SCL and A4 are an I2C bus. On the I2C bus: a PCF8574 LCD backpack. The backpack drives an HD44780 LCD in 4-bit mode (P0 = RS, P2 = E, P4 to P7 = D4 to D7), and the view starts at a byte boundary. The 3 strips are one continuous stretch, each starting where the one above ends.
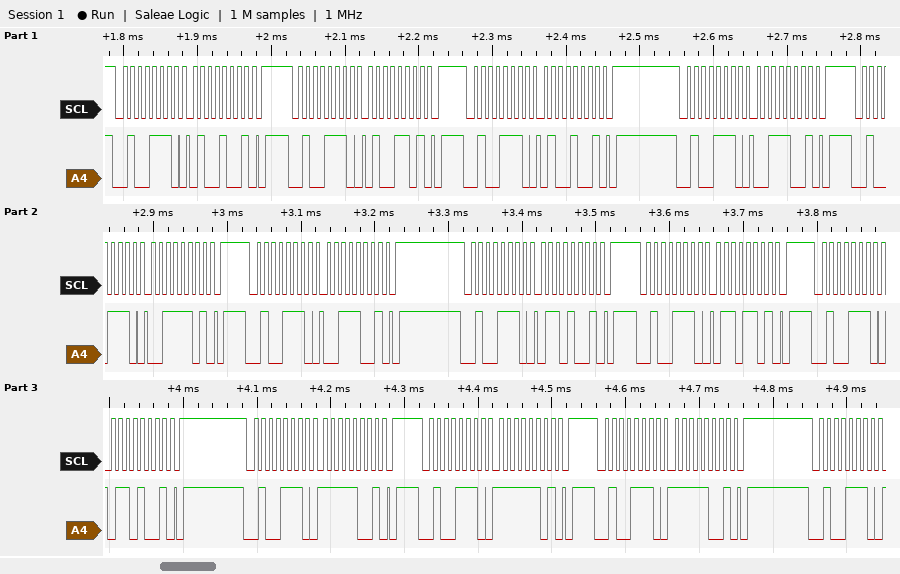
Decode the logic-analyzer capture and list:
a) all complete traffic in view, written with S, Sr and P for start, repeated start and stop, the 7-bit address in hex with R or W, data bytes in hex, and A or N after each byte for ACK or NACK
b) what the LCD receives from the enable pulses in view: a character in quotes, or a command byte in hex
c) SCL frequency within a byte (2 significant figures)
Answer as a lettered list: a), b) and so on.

a) S 27W A 49 A P S 27W A 4D A P S 27W A 49 A P S 27W A 39 A P S 27W A 3D A P S 27W A 39 A P S 27W A 69 A P S 27W A 6D A P S 27W A 69 A P S 27W A F9 A P S 27W A FD A P S 27W A F9 A P S 27W A
b) 'C' 'o'
c) 100 kHz
